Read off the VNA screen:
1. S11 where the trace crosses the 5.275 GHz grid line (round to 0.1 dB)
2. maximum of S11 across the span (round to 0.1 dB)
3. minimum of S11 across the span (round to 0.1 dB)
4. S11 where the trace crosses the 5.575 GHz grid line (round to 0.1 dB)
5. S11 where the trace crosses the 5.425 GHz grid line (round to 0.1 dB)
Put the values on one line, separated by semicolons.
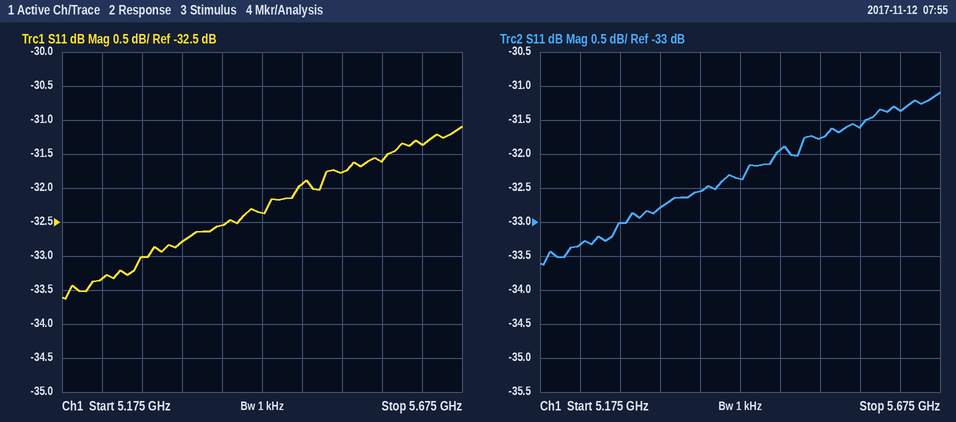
-33.0 dB; -31.1 dB; -33.6 dB; -31.6 dB; -32.4 dB
